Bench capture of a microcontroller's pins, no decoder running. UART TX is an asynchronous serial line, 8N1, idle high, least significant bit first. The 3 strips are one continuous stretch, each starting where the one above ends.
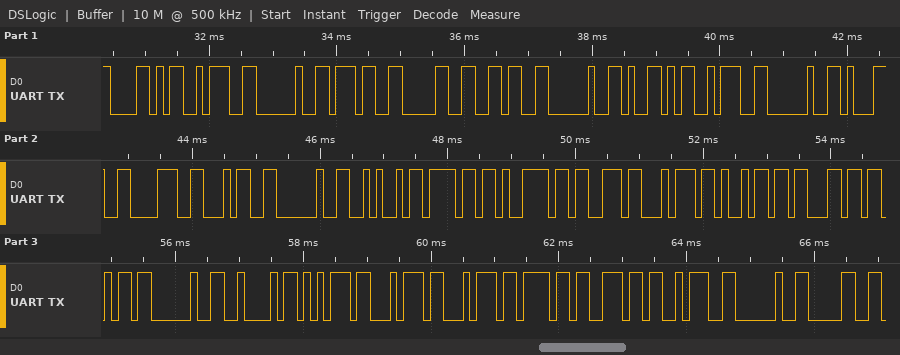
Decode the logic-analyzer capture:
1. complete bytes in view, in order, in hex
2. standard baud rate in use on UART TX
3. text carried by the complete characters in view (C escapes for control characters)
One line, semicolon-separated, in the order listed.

58 3A 20 37 30 36 20 59 3A 20 31 38 34 20 4A 6F 79 73 74 69 63 6B 20 42 75 74 74 6F 6E 3A 20 30; 9600 baud; "X: 706 Y: 184 Joystick Button: 0"
